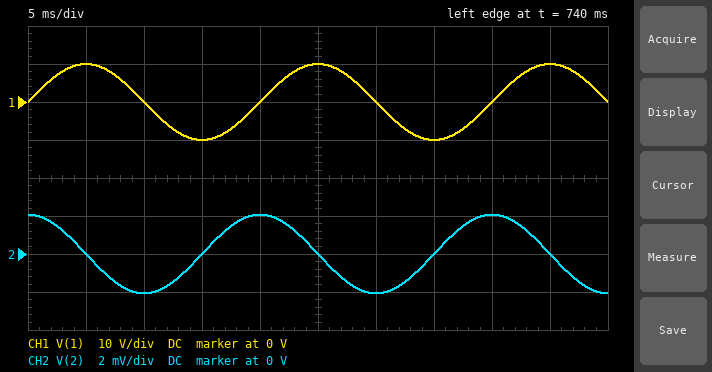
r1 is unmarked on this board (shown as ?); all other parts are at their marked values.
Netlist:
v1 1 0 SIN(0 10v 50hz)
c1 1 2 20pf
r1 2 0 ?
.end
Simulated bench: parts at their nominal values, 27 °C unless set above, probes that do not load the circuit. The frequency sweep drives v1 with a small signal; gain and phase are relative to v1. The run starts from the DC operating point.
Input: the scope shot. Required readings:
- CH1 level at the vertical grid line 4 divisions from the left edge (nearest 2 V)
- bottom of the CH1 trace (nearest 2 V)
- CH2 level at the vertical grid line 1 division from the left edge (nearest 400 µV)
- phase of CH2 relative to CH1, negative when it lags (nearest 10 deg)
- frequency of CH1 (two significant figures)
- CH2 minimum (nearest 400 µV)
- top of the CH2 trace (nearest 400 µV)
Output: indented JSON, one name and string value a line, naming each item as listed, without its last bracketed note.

{
  "CH1 level at the vertical grid line 4 divisions from the left edge": "0 V",
  "bottom of the CH1 trace": "-10 V",
  "CH2 level at the vertical grid line 1 division from the left edge": "0 V",
  "phase of CH2 relative to CH1, negative when it lags": "90 deg",
  "frequency of CH1": "50 Hz",
  "CH2 minimum": "-2.0 mV",
  "top of the CH2 trace": "2.0 mV"
}
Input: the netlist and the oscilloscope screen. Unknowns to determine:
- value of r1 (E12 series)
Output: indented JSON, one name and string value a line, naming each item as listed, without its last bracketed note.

{
  "value of r1": "33 kΩ"
}
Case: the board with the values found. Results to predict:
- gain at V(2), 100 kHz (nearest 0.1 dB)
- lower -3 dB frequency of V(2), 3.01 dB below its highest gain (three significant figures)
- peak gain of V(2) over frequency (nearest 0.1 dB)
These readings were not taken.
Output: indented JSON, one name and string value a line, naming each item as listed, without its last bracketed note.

{
  "gain at V(2), 100 kHz": "-8.3 dB",
  "lower -3 dB frequency of V(2), 3.01 dB below its highest gain": "241 kHz",
  "peak gain of V(2) over frequency": "0 dB"
}
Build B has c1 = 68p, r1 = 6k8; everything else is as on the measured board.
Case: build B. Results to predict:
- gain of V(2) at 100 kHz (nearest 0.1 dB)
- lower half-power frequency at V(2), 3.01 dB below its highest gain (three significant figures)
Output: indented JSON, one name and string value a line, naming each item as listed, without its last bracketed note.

{
  "gain of V(2) at 100 kHz": "-11.1 dB",
  "lower half-power frequency at V(2), 3.01 dB below its highest gain": "344 kHz"
}
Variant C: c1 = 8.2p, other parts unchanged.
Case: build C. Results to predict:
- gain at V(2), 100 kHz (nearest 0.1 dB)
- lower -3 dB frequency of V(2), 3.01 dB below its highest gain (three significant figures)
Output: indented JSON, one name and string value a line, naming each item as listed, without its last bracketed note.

{
  "gain at V(2), 100 kHz": "-15.5 dB",
  "lower -3 dB frequency of V(2), 3.01 dB below its highest gain": "588 kHz"
}
